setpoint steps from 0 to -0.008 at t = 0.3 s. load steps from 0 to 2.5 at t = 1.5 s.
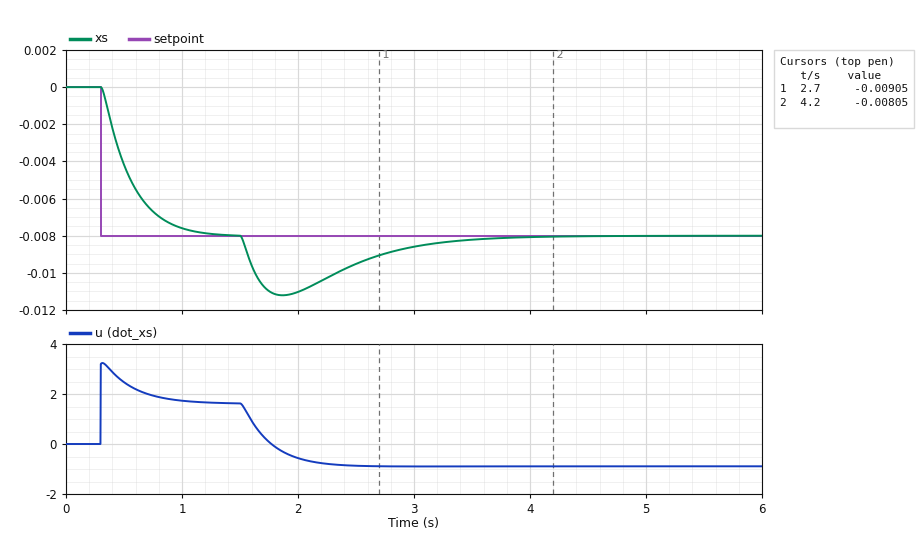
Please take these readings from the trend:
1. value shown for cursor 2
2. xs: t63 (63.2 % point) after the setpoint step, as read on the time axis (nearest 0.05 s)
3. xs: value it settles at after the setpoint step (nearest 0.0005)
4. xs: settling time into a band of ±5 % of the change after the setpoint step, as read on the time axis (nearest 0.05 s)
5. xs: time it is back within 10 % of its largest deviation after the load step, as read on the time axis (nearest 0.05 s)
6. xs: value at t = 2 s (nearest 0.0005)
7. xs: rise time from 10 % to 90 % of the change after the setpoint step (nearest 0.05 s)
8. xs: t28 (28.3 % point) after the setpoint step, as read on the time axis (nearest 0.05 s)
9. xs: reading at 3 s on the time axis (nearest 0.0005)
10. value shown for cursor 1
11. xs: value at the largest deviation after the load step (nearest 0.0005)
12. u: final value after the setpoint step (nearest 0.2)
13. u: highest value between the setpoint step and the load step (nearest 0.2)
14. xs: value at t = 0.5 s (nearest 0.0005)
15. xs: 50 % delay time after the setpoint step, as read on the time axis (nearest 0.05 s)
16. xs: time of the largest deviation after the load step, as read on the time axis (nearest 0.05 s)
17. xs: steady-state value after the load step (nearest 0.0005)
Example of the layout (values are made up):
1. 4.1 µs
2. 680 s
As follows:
1. -0.00805
2. 0.55 s
3. -0.0080
4. 1.00 s
5. 3.30 s
6. -0.0110
7. 0.50 s
8. 0.40 s
9. -0.0085
10. -0.00905
11. -0.0110
12. 1.6
13. 3.2
14. -0.0040
15. 0.50 s
16. 1.85 s
17. -0.0080
